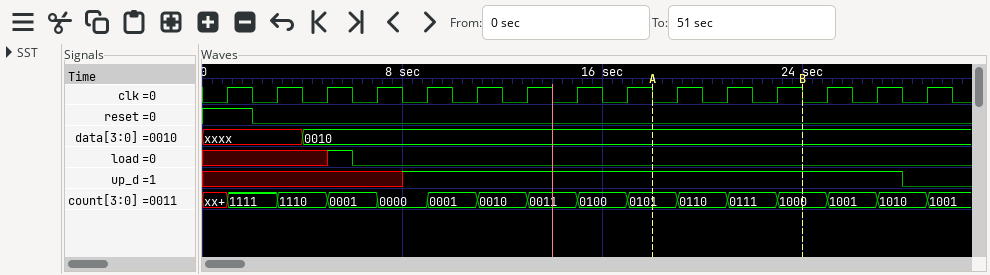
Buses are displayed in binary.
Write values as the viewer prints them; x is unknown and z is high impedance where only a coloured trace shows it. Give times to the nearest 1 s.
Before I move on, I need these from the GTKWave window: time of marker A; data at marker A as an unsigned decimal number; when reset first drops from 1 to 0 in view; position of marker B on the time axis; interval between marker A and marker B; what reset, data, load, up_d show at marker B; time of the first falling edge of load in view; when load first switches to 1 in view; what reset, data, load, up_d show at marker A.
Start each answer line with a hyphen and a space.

- 18 s
- 2
- 2 s
- 24 s
- 6 s
- reset=0, data=0010, load=0, up_d=1
- 6 s
- 5 s
- reset=0, data=0010, load=0, up_d=1
